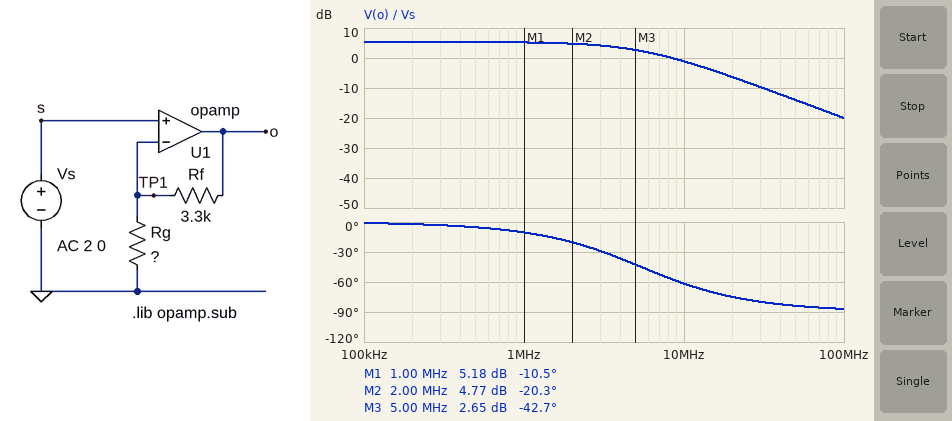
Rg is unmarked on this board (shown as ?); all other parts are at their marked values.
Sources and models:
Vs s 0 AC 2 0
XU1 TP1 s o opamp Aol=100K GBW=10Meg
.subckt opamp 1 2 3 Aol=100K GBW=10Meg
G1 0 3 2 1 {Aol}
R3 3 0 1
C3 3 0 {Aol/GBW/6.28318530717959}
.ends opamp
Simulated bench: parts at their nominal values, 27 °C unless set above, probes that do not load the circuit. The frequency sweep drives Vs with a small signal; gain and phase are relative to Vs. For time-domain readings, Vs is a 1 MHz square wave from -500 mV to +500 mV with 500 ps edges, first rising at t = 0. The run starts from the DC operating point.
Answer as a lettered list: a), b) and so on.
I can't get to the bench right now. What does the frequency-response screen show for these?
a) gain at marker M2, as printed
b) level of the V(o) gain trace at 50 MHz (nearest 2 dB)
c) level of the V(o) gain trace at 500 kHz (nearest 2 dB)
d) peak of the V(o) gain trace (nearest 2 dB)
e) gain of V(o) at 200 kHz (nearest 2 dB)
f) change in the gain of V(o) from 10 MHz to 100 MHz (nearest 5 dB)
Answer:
a) 4.77 dB
b) -14 dB
c) 6 dB
d) 6 dB
e) 6 dB
f) -20 dB
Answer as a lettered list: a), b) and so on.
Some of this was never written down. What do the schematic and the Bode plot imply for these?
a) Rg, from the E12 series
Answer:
a) 3.9 kΩ
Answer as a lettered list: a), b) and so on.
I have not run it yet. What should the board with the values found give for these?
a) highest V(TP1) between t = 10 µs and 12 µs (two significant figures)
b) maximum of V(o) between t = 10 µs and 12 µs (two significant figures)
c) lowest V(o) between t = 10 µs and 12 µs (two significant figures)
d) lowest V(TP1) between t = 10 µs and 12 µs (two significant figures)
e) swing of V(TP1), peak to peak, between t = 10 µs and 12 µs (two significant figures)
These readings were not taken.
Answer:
a) 500 mV
b) 920 mV
c) -920 mV
d) -500 mV
e) 1.0 V
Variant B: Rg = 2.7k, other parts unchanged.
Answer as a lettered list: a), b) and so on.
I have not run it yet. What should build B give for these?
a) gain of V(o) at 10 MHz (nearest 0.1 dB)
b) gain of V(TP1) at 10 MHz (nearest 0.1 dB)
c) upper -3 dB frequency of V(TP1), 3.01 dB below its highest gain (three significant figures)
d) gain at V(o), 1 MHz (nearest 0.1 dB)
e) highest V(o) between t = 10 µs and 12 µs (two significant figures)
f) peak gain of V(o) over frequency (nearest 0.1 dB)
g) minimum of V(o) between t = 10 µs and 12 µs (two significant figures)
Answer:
a) -0.8 dB
b) -7.7 dB
c) 4.50 MHz
d) 6.7 dB
e) 1.1 V
f) 6.9 dB
g) -1.1 V
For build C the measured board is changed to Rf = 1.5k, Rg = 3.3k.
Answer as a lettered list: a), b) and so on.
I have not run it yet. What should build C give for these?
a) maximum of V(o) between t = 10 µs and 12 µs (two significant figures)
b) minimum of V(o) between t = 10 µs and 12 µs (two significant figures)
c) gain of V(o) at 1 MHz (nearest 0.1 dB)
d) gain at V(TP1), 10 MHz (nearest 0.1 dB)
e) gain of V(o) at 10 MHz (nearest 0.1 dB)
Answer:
a) 730 mV
b) -730 mV
c) 3.2 dB
d) -4.9 dB
e) -1.7 dB
